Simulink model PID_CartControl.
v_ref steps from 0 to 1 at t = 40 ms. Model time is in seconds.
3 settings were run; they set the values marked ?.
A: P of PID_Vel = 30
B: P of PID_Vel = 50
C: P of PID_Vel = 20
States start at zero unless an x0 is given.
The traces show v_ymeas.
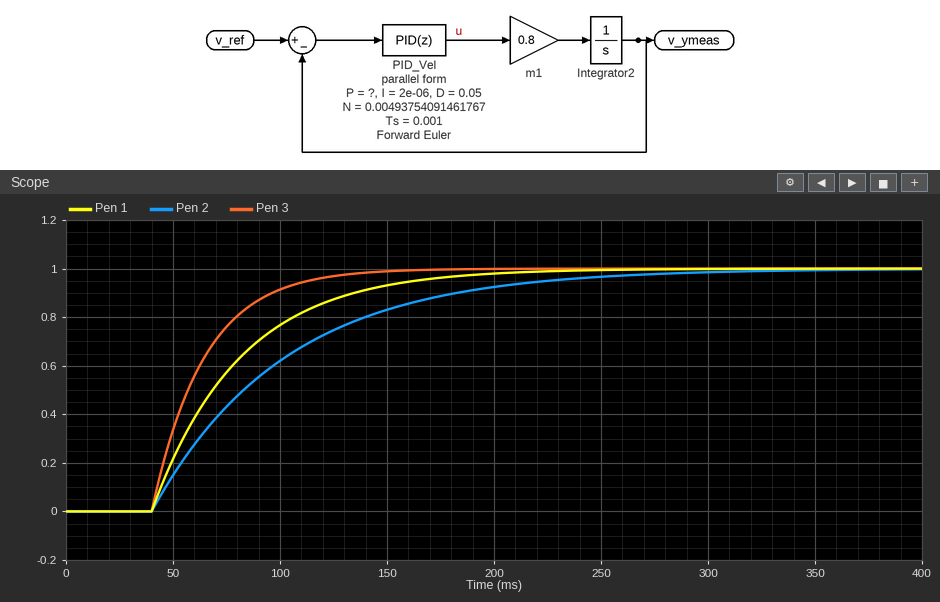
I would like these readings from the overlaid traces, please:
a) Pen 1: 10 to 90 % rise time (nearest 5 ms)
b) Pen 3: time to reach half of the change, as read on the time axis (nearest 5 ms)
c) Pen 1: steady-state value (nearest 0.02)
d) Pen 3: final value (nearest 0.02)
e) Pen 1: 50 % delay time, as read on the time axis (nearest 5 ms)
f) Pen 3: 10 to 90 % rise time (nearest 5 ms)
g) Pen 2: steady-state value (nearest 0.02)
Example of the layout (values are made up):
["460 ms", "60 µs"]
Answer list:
["90 ms", "55 ms", "1.00", "1.00", "70 ms", "55 ms", "1.00"]
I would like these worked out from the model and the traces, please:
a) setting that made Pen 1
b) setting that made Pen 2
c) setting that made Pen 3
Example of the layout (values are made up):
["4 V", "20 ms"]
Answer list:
["A", "C", "B"]
